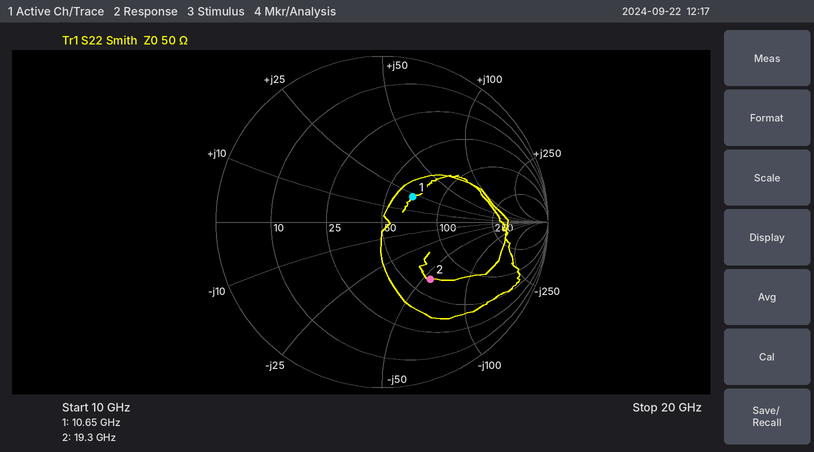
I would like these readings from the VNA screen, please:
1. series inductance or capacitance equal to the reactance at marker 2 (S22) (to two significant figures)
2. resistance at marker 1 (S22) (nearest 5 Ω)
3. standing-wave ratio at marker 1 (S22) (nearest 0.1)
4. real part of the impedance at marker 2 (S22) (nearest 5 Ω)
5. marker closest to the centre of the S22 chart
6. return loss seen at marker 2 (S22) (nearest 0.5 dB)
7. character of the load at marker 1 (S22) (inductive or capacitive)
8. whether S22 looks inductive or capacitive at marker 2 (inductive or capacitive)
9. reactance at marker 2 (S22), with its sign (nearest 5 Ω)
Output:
150 fF
70 Ω
1.6
65 Ω
marker 1
7.0 dB
inductive
capacitive
-55 Ω
